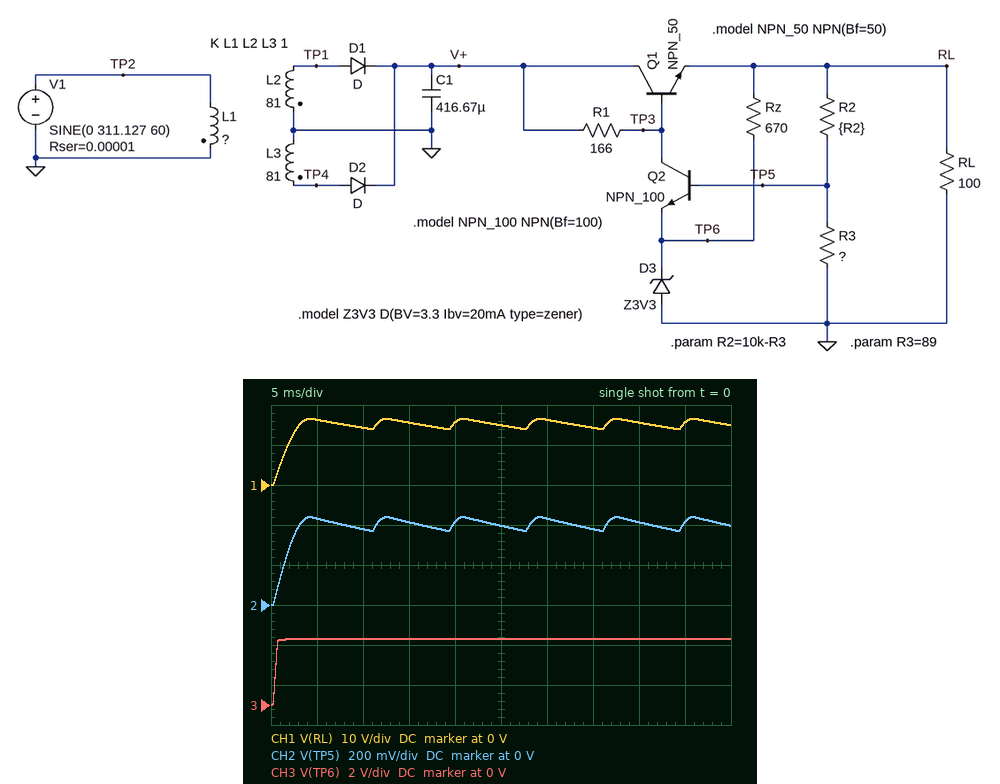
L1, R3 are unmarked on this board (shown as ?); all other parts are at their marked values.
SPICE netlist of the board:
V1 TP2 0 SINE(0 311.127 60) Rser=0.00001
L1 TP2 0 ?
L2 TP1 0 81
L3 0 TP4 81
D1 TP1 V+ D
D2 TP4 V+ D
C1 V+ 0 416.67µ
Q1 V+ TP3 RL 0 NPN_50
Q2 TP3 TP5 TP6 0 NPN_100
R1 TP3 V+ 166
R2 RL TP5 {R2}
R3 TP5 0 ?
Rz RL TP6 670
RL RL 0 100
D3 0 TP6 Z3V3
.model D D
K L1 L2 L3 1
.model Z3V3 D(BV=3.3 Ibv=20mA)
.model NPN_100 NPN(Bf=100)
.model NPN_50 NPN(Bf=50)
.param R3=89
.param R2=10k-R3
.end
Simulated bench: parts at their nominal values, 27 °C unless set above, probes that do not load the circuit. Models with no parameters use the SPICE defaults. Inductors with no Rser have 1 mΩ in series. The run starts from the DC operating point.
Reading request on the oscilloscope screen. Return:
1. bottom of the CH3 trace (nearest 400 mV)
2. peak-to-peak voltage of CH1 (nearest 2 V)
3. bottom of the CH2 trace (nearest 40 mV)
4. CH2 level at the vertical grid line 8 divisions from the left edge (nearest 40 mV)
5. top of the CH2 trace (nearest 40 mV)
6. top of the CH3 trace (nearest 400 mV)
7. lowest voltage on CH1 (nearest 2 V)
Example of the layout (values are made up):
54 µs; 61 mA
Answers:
0 V; 16 V; 0 V; 400 mV; 440 mV; 3.2 V; 0 V
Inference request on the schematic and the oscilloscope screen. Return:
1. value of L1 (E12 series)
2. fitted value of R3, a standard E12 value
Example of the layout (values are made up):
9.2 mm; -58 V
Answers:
22 kH; 270 Ω
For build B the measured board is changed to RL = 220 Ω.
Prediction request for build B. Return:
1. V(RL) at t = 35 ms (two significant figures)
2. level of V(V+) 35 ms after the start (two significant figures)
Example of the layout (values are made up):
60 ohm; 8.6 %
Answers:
16 V; 17 V
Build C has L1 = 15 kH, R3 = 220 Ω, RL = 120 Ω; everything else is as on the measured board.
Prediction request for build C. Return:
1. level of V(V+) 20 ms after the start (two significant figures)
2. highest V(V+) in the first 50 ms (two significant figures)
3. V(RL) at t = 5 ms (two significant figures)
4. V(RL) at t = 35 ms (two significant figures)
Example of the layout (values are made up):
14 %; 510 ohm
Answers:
21 V; 22 V; 20 V; 18 V
